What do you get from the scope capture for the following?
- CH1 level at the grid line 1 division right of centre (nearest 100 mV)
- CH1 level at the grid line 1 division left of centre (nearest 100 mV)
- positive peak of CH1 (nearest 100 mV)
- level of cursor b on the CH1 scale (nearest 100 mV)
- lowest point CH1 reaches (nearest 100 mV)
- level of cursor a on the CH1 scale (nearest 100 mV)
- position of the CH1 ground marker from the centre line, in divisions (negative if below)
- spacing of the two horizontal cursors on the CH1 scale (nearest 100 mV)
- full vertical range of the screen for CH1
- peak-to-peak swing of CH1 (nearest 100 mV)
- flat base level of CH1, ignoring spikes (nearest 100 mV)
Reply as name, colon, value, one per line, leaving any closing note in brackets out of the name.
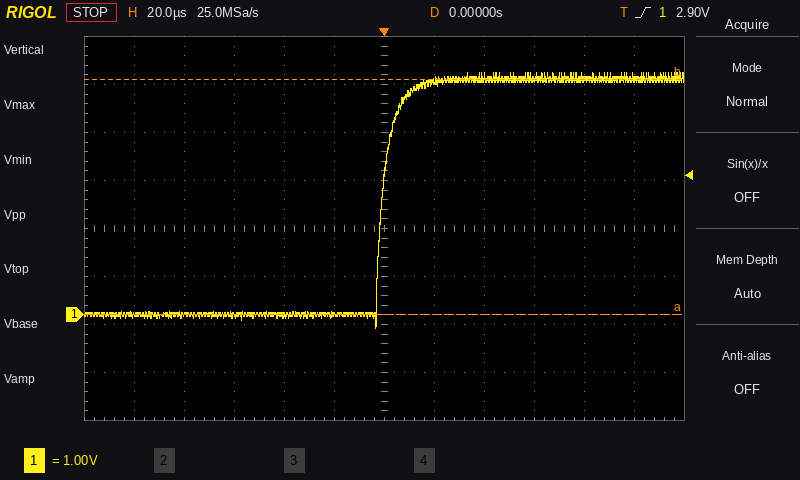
CH1 level at the grid line 1 division right of centre: 4.9 V
CH1 level at the grid line 1 division left of centre: 0.0 V
positive peak of CH1: 5.0 V
level of cursor b on the CH1 scale: 4.9 V
lowest point CH1 reaches: -300 mV
level of cursor a on the CH1 scale: 0.0 V
position of the CH1 ground marker from the centre line, in divisions: -1.8 div
spacing of the two horizontal cursors on the CH1 scale: 4.9 V
full vertical range of the screen for CH1: 8 V
peak-to-peak swing of CH1: 5.3 V
flat base level of CH1, ignoring spikes: 0.0 V
